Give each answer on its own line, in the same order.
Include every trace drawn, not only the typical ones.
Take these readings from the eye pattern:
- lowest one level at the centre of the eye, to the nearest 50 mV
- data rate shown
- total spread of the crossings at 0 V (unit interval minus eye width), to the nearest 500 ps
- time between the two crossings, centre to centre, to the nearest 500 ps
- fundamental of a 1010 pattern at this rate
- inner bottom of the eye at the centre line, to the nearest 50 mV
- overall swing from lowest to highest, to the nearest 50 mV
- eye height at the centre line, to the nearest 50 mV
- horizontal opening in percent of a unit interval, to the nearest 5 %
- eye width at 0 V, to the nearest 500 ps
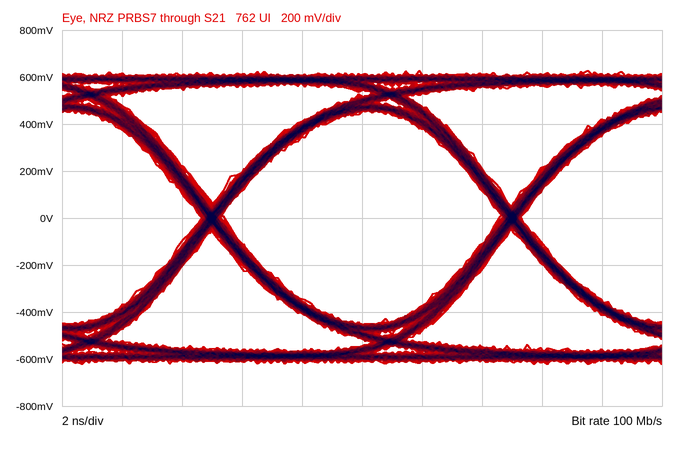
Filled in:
450 mV
100 Mb/s
1.0 ns
10.0 ns
50 MHz
-450 mV
1.25 V
900 mV
90 %
9.0 ns
